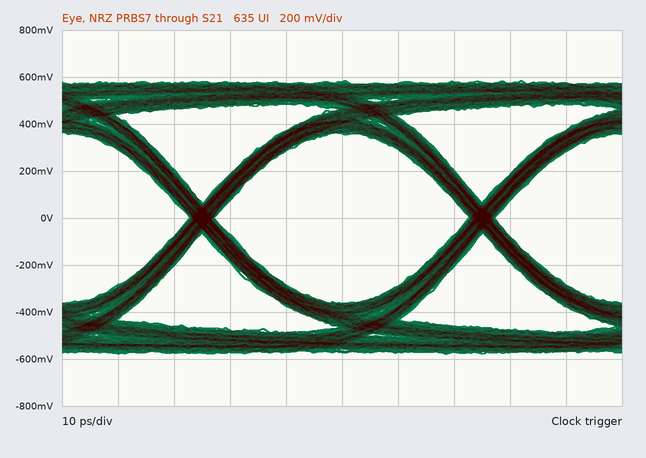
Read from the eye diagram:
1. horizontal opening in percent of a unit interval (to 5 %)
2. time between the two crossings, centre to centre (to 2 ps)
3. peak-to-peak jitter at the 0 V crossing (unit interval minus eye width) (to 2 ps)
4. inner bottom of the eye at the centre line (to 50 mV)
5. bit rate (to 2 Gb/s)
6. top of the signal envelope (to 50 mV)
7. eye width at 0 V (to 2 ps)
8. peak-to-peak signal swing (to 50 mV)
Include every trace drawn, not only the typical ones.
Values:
90 %
50 ps
4 ps
-350 mV
20 Gb/s
600 mV
46 ps
1.15 V
